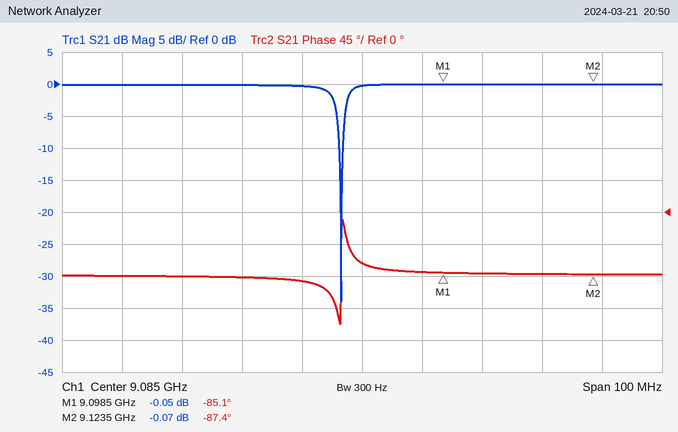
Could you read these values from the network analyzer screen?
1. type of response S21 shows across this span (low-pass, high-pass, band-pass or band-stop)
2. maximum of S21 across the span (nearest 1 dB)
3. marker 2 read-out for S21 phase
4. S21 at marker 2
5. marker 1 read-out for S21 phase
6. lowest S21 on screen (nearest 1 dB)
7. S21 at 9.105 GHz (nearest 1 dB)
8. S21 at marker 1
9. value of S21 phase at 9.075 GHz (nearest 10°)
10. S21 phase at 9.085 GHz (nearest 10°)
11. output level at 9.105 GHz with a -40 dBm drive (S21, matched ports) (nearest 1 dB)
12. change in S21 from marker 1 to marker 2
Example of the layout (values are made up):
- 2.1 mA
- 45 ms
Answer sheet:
- band-stop
- 0 dB
- -87.4°
- -0.07 dB
- -85.1°
- -34 dB
- 0 dB
- -0.05 dB
- -100°
- -70°
- -40 dBm
- -0.02 dB
